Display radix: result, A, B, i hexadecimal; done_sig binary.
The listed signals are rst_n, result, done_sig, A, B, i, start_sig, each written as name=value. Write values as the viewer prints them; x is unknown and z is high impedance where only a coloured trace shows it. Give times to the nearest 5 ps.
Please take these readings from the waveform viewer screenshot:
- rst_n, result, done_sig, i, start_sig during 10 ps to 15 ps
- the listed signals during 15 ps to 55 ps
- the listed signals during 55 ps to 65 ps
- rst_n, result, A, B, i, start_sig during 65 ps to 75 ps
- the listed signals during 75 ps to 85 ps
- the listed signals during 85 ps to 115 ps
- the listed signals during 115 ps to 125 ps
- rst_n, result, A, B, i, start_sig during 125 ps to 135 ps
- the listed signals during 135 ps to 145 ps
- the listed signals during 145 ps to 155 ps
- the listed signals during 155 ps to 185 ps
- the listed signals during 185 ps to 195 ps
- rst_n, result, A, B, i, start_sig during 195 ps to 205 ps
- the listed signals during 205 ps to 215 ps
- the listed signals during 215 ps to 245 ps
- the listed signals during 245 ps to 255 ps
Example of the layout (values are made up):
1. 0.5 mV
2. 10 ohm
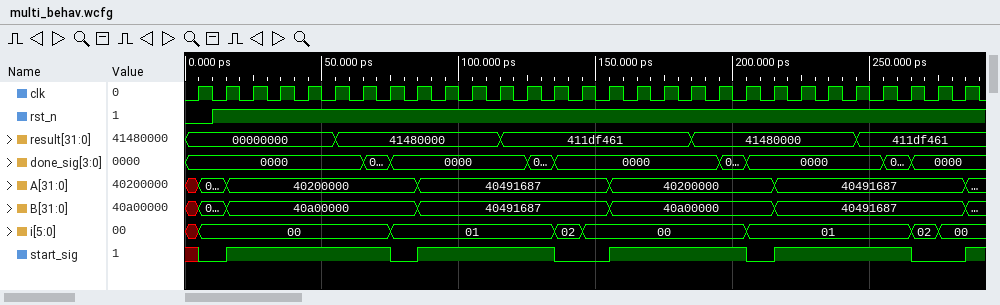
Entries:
1. rst_n=1, result=00000000, done_sig=0000, i=00, start_sig=0
2. rst_n=1, result=00000000, done_sig=0000, A=40200000, B=40a00000, i=00, start_sig=1
3. rst_n=1, result=41480000, done_sig=0000, A=40200000, B=40a00000, i=00, start_sig=1
4. rst_n=1, result=41480000, A=40200000, B=40a00000, i=00, start_sig=1
5. rst_n=1, result=41480000, done_sig=0000, A=40200000, B=40a00000, i=01, start_sig=0
6. rst_n=1, result=41480000, done_sig=0000, A=40491687, B=40491687, i=01, start_sig=1
7. rst_n=1, result=411df461, done_sig=0000, A=40491687, B=40491687, i=01, start_sig=1
8. rst_n=1, result=411df461, A=40491687, B=40491687, i=01, start_sig=1
9. rst_n=1, result=411df461, done_sig=0000, A=40491687, B=40491687, i=02, start_sig=0
10. rst_n=1, result=411df461, done_sig=0000, A=40491687, B=40491687, i=00, start_sig=0
11. rst_n=1, result=411df461, done_sig=0000, A=40200000, B=40a00000, i=00, start_sig=1
12. rst_n=1, result=41480000, done_sig=0000, A=40200000, B=40a00000, i=00, start_sig=1
13. rst_n=1, result=41480000, A=40200000, B=40a00000, i=00, start_sig=1
14. rst_n=1, result=41480000, done_sig=0000, A=40200000, B=40a00000, i=01, start_sig=0
15. rst_n=1, result=41480000, done_sig=0000, A=40491687, B=40491687, i=01, start_sig=1
16. rst_n=1, result=411df461, done_sig=0000, A=40491687, B=40491687, i=01, start_sig=1
